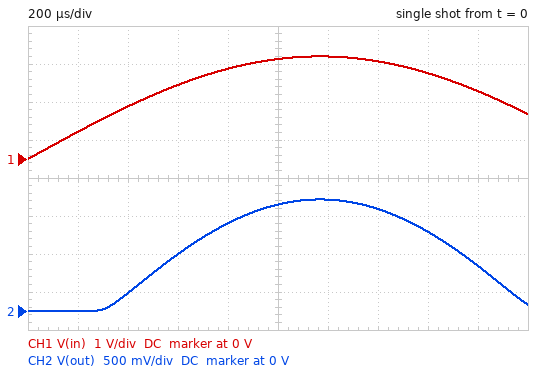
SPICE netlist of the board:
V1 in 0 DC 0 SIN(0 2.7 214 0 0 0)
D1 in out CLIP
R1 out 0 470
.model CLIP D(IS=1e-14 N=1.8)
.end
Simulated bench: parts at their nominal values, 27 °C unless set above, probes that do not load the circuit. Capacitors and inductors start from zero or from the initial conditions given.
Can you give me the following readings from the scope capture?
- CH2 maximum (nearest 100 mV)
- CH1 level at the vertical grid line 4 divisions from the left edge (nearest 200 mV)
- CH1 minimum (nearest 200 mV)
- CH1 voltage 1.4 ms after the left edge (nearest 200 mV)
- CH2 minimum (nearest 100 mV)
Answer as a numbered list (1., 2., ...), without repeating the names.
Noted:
1. 1.5 V
2. 2.4 V
3. 0 V
4. 2.6 V
5. 0 V
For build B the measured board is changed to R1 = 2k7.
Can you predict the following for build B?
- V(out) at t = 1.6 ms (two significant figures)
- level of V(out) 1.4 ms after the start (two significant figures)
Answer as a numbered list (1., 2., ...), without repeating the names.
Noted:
1. 1.1 V
2. 1.4 V
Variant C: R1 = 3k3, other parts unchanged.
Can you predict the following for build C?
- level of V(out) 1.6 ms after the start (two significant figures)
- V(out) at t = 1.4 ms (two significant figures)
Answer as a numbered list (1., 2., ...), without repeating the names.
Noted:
1. 1.1 V
2. 1.4 V
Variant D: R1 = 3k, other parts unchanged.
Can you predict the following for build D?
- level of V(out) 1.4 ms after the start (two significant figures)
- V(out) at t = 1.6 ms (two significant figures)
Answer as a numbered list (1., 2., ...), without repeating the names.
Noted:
1. 1.4 V
2. 1.1 V
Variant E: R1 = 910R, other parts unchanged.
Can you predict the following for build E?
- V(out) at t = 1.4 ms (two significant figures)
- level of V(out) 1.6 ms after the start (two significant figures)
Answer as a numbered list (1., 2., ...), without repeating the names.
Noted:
1. 1.4 V
2. 1.1 V
